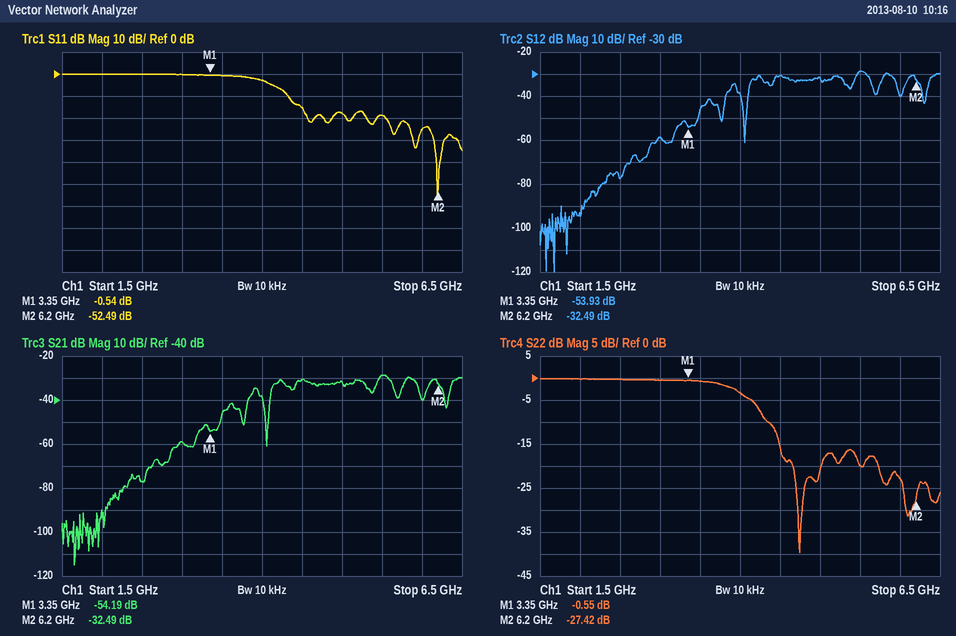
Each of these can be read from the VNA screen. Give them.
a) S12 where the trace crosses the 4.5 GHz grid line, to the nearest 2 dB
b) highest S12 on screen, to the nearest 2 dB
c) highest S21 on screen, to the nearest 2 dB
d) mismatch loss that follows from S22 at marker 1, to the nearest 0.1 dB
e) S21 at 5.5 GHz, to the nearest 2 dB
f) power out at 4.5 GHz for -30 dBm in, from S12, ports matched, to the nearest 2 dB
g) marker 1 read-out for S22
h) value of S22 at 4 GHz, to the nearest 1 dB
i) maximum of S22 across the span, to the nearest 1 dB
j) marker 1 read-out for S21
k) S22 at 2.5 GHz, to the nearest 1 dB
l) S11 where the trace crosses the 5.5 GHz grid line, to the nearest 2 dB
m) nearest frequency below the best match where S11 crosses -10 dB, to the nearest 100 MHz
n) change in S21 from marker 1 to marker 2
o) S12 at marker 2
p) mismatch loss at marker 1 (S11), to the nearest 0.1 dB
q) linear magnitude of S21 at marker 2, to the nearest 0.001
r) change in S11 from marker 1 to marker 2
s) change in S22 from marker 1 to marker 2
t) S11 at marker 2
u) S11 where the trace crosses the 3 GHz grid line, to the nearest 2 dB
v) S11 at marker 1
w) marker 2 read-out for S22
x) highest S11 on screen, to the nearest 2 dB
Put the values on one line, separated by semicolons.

-30 dB; -28 dB; -28 dB; 9.2 dB; -28 dB; -60 dBm; -0.55 dB; -3 dB; 0 dB; -54.19 dB; 0 dB; -18 dB; 4.3 GHz; 21.70 dB; -32.49 dB; 9.3 dB; 0.024; -51.95 dB; -26.87 dB; -52.49 dB; 0 dB; -0.54 dB; -27.42 dB; 0 dB
